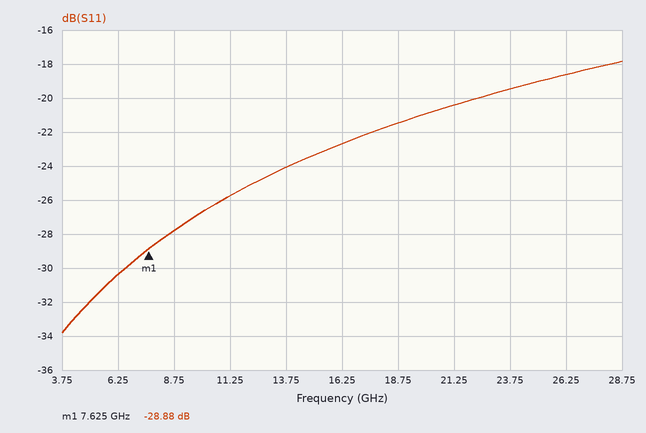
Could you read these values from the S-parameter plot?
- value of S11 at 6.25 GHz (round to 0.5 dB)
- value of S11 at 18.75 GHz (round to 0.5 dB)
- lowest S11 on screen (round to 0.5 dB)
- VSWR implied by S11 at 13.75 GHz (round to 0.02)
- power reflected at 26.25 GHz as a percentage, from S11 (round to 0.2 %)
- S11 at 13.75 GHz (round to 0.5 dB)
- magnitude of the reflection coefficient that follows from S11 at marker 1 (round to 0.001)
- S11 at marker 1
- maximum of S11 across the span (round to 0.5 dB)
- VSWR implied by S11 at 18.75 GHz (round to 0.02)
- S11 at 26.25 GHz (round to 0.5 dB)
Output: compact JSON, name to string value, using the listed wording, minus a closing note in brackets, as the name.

{"value of S11 at 6.25 GHz": "-30.5 dB", "value of S11 at 18.75 GHz": "-21.5 dB", "lowest S11 on screen": "-34.0 dB", "VSWR implied by S11 at 13.75 GHz": "1.14", "power reflected at 26.25 GHz as a percentage, from S11": "1.4 %", "S11 at 13.75 GHz": "-24.0 dB", "magnitude of the reflection coefficient that follows from S11 at marker 1": "0.036", "S11 at marker 1": "-28.88 dB", "maximum of S11 across the span": "-18.0 dB", "VSWR implied by S11 at 18.75 GHz": "1.18", "S11 at 26.25 GHz": "-18.5 dB"}
